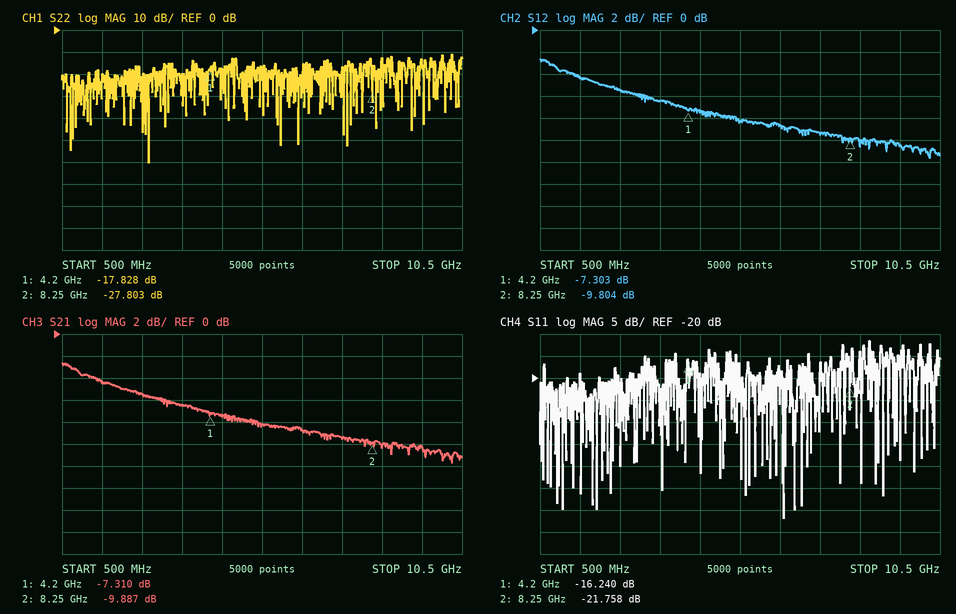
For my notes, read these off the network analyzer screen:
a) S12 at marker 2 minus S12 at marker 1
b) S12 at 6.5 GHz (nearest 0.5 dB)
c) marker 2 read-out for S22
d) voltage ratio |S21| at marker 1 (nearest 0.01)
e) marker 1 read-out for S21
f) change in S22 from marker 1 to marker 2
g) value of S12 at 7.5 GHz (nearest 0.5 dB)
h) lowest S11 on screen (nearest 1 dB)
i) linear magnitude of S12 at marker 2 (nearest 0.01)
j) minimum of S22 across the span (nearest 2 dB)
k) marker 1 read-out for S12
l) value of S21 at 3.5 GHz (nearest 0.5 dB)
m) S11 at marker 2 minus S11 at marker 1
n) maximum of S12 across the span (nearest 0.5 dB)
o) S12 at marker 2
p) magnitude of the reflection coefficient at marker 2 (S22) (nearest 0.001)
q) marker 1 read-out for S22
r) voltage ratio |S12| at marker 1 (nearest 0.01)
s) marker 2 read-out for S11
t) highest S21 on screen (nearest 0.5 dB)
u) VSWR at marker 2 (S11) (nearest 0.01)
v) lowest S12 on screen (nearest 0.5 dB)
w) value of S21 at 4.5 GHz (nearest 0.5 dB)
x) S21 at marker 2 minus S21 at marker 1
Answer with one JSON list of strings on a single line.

["-2.501 dB", "-8.5 dB", "-27.803 dB", "0.43", "-7.310 dB", "-9.975 dB", "-9.5 dB", "-52 dB", "0.32", "-60 dB", "-7.303 dB", "-6.5 dB", "-5.518 dB", "-2.5 dB", "-9.804 dB", "0.041", "-17.828 dB", "0.43", "-21.758 dB", "-2.5 dB", "1.18", "-11.5 dB", "-7.5 dB", "-2.577 dB"]
